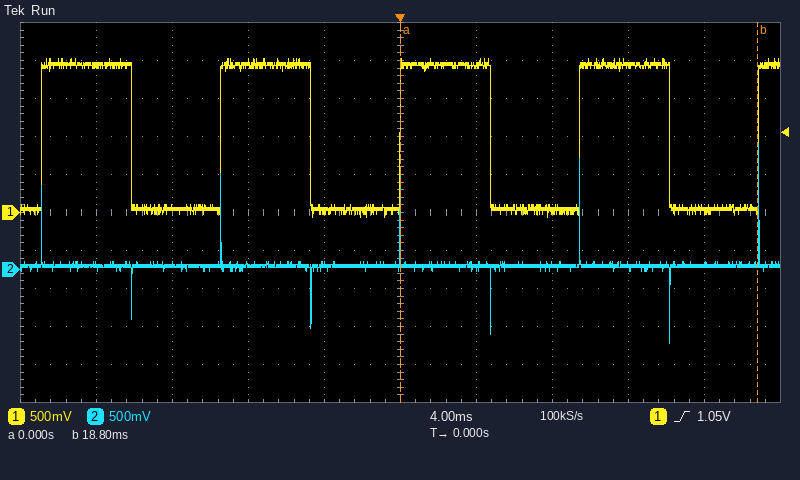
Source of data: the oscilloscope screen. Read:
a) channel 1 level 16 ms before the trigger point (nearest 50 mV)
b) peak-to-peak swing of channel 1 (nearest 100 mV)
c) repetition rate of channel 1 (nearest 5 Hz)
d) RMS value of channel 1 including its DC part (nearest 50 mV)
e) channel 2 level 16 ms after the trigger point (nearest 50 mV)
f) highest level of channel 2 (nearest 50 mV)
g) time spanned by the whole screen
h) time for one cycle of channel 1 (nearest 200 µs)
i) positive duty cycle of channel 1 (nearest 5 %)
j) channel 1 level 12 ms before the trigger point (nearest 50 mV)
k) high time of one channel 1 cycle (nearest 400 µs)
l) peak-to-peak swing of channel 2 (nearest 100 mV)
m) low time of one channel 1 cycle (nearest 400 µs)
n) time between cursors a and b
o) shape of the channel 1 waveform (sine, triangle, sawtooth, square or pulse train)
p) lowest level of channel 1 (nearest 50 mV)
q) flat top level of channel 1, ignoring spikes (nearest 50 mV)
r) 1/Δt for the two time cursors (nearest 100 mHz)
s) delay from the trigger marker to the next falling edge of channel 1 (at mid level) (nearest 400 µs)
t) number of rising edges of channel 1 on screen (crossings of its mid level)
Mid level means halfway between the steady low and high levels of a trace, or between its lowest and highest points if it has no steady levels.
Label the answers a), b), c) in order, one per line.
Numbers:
a) 1.95 V
b) 2.10 V
c) 105 Hz
d) 1.40 V
e) 50 mV
f) 1.65 V
g) 40 ms
h) 9.4 ms
i) 50 %
j) 50 mV
k) 4.8 ms
l) 2.60 V
m) 4.8 ms
n) 18.8 ms
o) square
p) -50 mV
q) 1.95 V
r) 53.2 Hz
s) 4.8 ms
t) 5
